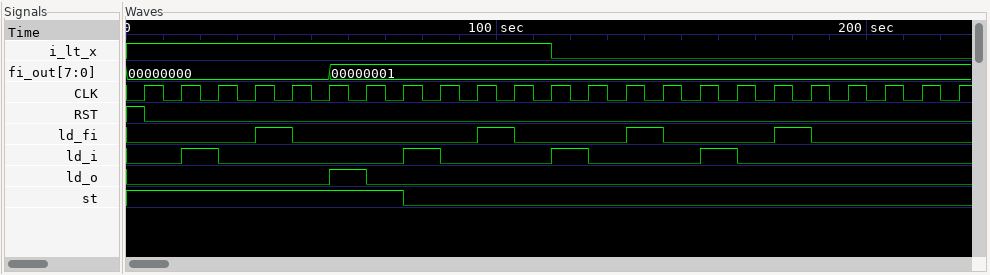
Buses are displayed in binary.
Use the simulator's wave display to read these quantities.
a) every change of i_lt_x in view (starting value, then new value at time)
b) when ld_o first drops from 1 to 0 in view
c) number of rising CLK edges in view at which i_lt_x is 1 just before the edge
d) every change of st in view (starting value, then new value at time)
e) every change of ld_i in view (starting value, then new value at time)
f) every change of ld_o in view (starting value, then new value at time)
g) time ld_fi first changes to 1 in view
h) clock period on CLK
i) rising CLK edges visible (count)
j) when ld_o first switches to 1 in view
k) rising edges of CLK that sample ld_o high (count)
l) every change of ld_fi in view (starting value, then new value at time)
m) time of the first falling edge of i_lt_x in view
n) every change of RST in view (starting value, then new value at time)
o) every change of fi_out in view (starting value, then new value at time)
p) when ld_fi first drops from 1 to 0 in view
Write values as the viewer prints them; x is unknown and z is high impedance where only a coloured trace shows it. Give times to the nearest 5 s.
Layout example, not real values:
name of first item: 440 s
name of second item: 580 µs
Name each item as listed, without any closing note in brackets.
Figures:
every change of i_lt_x in view: 1, 0 at 115 s
when ld_o first drops from 1 to 0 in view: 65 s
number of rising CLK edges in view at which i_lt_x is 1 just before the edge: 12
every change of st in view: 1, 0 at 75 s
every change of ld_i in view: 0, 1 at 15 s, 0 at 25 s, 1 at 75 s, 0 at 85 s, 1 at 115 s, 0 at 125 s, 1 at 155 s, 0 at 165 s
every change of ld_o in view: 0, 1 at 55 s, 0 at 65 s
time ld_fi first changes to 1 in view: 35 s
clock period on CLK: 10 s
rising CLK edges visible: 23
when ld_o first switches to 1 in view: 55 s
rising edges of CLK that sample ld_o high: 1
every change of ld_fi in view: 0, 1 at 35 s, 0 at 45 s, 1 at 95 s, 0 at 105 s, 1 at 135 s, 0 at 145 s, 1 at 175 s, 0 at 185 s
time of the first falling edge of i_lt_x in view: 115 s
every change of RST in view: 1, 0 at 5 s
every change of fi_out in view: 00000000, 00000001 at 55 s
when ld_fi first drops from 1 to 0 in view: 45 s
